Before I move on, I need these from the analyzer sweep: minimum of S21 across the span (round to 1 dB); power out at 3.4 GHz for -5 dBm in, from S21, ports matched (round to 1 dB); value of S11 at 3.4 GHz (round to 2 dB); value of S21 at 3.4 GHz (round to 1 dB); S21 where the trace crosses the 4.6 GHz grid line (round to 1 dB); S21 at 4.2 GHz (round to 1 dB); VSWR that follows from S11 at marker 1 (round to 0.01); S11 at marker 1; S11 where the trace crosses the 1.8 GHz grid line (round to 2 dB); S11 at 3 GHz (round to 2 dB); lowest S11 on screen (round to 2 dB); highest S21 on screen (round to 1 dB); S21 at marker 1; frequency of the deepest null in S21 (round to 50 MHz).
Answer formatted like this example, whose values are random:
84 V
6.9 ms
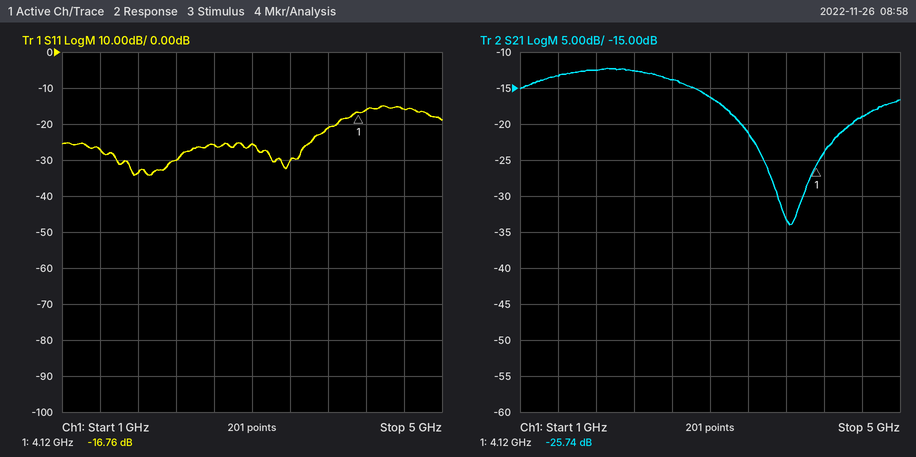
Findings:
-34 dB
-26 dBm
-30 dB
-21 dB
-19 dB
-24 dB
1.34
-16.76 dB
-34 dB
-26 dB
-34 dB
-12 dB
-25.74 dB
3.85 GHz
